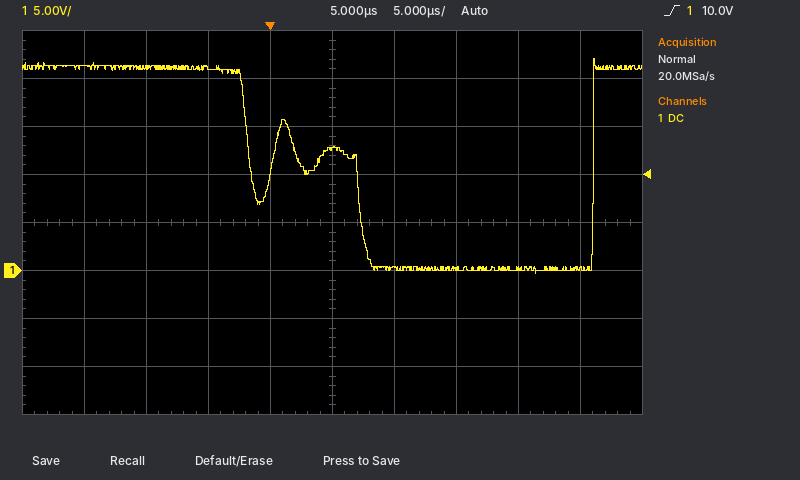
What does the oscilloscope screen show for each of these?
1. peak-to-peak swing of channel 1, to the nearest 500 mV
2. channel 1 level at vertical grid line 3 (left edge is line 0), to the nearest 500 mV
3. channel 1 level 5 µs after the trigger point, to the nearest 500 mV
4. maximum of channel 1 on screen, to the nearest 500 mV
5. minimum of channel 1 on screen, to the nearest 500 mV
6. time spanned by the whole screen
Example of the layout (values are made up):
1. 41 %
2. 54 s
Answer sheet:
1. 22.5 V
2. 21.0 V
3. 12.5 V
4. 22.0 V
5. -500 mV
6. 50 µs
